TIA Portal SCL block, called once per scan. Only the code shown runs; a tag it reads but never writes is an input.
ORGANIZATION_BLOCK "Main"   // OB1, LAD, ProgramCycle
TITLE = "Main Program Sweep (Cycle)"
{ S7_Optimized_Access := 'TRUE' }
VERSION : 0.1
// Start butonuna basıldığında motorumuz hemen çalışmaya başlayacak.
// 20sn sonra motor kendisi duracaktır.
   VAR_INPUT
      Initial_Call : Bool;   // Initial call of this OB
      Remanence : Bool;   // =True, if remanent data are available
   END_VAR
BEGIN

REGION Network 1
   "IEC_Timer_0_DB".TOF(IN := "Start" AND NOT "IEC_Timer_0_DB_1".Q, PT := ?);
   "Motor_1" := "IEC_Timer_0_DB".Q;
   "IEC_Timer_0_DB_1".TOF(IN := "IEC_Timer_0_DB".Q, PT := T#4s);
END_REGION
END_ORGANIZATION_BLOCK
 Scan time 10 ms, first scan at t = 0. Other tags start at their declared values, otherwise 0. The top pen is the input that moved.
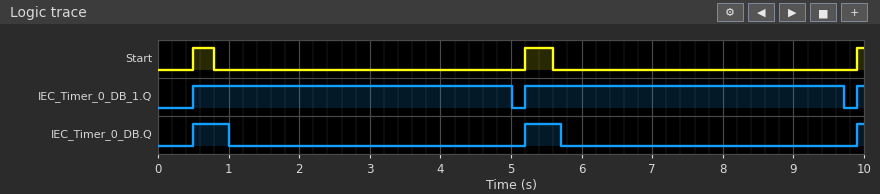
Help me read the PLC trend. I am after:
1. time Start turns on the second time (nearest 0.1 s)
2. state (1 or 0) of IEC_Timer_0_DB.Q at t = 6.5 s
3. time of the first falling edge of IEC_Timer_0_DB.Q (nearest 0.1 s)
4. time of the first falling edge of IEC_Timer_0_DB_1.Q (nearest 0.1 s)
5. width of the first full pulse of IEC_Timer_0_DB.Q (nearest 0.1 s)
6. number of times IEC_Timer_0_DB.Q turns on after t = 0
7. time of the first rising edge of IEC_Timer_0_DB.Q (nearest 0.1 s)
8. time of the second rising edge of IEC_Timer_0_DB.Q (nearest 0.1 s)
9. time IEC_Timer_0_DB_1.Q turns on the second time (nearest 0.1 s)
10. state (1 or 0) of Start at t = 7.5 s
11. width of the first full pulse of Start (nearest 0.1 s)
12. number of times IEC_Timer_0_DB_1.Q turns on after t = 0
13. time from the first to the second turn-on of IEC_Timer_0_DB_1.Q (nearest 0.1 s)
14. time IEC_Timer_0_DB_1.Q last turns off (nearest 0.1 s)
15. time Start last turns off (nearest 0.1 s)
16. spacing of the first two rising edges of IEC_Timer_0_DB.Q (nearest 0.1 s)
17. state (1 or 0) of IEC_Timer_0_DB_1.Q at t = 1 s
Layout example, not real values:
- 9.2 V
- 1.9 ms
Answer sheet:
- 5.2 s
- 0
- 1.0 s
- 5.0 s
- 0.5 s
- 3
- 0.5 s
- 5.2 s
- 5.2 s
- 0
- 0.3 s
- 3
- 4.7 s
- 9.7 s
- 5.6 s
- 4.7 s
- 1
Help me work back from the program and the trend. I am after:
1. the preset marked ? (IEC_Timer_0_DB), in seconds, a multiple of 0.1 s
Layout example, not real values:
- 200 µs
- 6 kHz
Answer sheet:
- 0.5 s
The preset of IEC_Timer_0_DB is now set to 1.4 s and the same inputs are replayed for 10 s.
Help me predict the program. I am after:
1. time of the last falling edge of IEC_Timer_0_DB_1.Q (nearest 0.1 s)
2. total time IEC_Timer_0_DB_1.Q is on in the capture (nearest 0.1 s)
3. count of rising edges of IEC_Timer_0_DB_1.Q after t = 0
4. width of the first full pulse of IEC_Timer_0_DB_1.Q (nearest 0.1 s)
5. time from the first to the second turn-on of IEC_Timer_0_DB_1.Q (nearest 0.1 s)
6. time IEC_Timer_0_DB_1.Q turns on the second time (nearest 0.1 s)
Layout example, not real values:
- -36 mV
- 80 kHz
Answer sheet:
- 5.9 s
- 5.5 s
- 2
- 5.4 s
- 9.4 s
- 9.9 s
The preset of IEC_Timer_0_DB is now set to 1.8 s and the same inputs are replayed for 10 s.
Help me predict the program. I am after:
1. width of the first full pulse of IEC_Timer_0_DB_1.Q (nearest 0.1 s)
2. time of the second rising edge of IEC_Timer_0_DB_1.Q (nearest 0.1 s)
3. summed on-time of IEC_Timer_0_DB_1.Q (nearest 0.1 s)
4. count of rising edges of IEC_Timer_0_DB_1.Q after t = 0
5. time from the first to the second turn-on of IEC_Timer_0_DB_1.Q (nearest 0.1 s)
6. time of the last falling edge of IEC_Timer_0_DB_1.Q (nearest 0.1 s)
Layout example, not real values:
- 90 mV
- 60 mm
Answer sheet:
- 5.8 s
- 9.9 s
- 5.9 s
- 2
- 9.4 s
- 6.3 s
